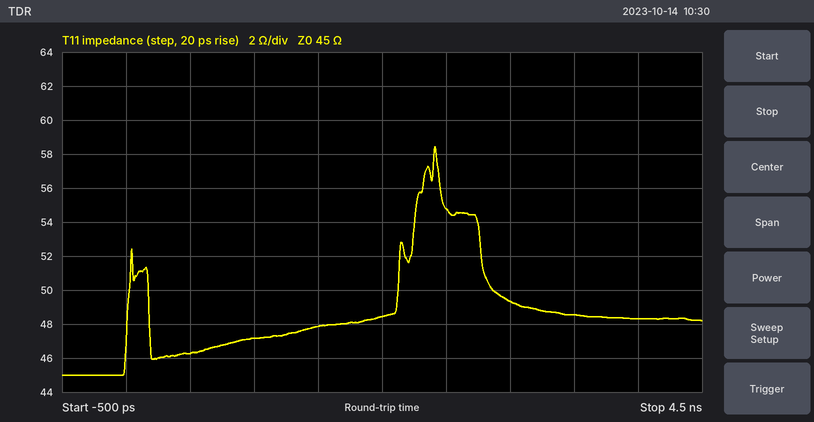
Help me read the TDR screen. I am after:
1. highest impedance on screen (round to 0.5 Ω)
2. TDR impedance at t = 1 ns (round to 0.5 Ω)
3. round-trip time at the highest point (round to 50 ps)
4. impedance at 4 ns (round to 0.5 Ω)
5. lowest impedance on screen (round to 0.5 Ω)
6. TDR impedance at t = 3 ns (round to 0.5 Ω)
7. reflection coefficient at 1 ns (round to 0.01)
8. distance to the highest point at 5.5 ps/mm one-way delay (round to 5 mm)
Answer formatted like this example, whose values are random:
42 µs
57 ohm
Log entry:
58.5 Ω
47.0 Ω
2.40 ns
48.5 Ω
45.0 Ω
49.5 Ω
+0.02
220 mm
